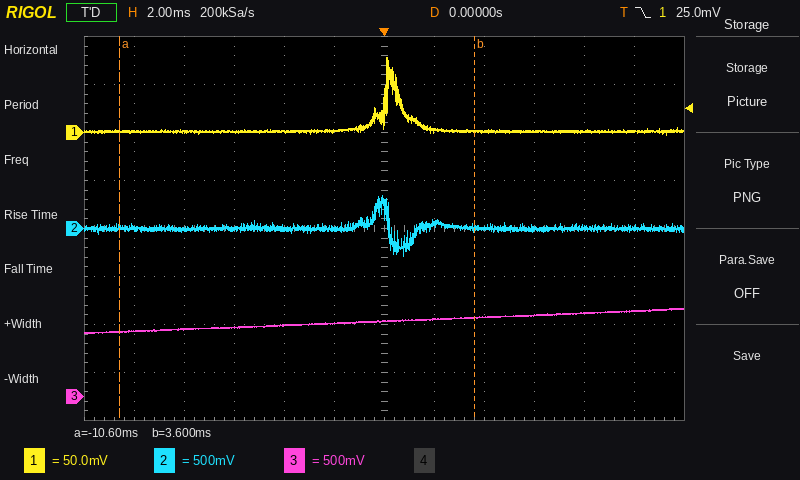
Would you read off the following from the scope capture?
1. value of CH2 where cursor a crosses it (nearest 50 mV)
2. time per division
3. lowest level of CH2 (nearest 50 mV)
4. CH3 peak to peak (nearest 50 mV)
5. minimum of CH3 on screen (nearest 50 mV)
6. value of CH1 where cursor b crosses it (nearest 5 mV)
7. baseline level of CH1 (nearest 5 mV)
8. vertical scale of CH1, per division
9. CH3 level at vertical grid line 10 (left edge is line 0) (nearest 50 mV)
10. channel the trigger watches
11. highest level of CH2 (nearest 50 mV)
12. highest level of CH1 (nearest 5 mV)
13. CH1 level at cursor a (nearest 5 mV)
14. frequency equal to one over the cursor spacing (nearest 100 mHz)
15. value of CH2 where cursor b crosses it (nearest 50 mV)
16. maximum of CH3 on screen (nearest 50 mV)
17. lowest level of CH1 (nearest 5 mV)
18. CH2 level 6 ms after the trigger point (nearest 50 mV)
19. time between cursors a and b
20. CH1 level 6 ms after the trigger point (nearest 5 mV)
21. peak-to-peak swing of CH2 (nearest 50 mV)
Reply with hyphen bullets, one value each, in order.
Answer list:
- 0 mV
- 2 ms
- -300 mV
- 250 mV
- 650 mV
- 0 mV
- 0 mV
- 50 mV
- 850 mV
- CH1
- 350 mV
- 80 mV
- 0 mV
- 70.4 Hz
- 0 mV
- 900 mV
- -5 mV
- 0 mV
- 14.2 ms
- 0 mV
- 650 mV
